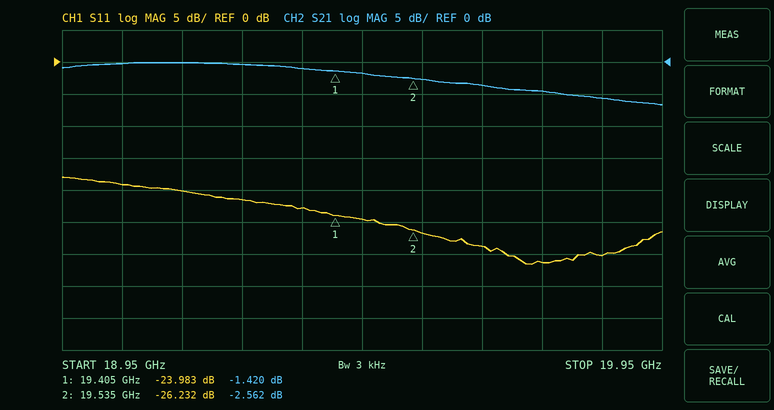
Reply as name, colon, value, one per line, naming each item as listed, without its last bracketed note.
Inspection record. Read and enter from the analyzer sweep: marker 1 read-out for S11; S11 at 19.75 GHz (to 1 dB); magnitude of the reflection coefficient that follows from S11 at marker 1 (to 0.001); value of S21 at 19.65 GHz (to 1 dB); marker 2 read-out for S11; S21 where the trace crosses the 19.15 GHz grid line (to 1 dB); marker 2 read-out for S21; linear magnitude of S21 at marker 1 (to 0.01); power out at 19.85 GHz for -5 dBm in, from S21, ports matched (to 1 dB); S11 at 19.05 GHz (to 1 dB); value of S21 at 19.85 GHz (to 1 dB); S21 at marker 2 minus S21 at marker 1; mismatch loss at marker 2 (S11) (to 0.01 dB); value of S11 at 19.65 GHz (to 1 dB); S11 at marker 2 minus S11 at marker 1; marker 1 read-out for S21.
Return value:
marker 1 read-out for S11: -23.983 dB
S11 at 19.75 GHz: -31 dB
magnitude of the reflection coefficient that follows from S11 at marker 1: 0.063
value of S21 at 19.65 GHz: -4 dB
marker 2 read-out for S11: -26.232 dB
S21 where the trace crosses the 19.15 GHz grid line: 0 dB
marker 2 read-out for S21: -2.562 dB
linear magnitude of S21 at marker 1: 0.85
power out at 19.85 GHz for -5 dBm in, from S21, ports matched: -11 dBm
S11 at 19.05 GHz: -19 dB
value of S21 at 19.85 GHz: -6 dB
S21 at marker 2 minus S21 at marker 1: -1.142 dB
mismatch loss at marker 2 (S11): 0.01 dB
value of S11 at 19.65 GHz: -29 dB
S11 at marker 2 minus S11 at marker 1: -2.249 dB
marker 1 read-out for S21: -1.420 dB
